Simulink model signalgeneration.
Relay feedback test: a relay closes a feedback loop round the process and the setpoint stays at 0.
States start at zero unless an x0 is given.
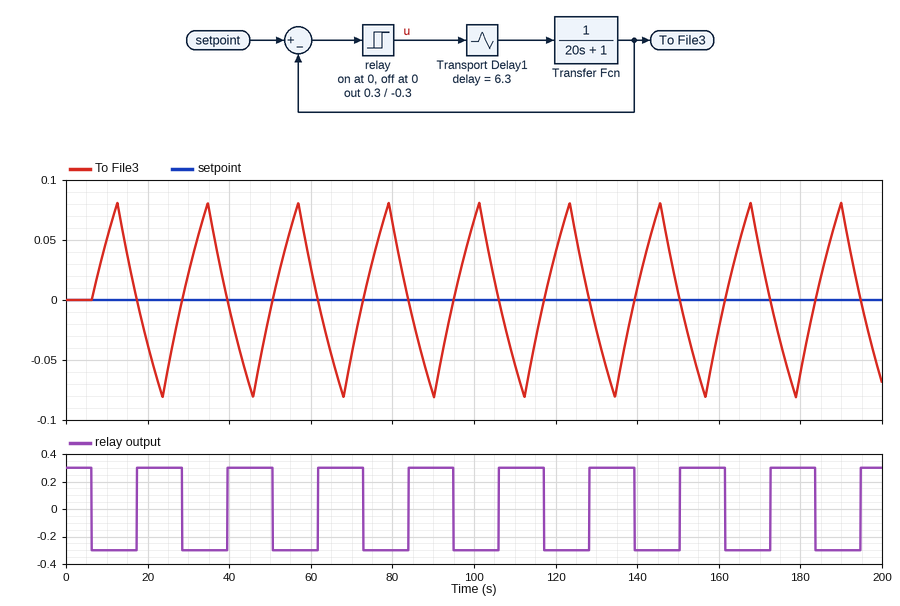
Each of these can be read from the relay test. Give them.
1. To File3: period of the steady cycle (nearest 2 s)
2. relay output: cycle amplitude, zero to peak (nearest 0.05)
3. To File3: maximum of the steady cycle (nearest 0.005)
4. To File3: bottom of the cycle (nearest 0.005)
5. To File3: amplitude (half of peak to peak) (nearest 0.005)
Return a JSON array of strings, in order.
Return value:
["22 s", "0.30", "0.080", "-0.080", "0.080"]
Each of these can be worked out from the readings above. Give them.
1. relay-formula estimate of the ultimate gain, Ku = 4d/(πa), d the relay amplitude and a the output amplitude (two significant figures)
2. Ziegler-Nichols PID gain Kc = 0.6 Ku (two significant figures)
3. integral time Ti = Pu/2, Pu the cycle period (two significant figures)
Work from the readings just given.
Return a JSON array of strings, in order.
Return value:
["4.8", "2.9", "11 s"]
